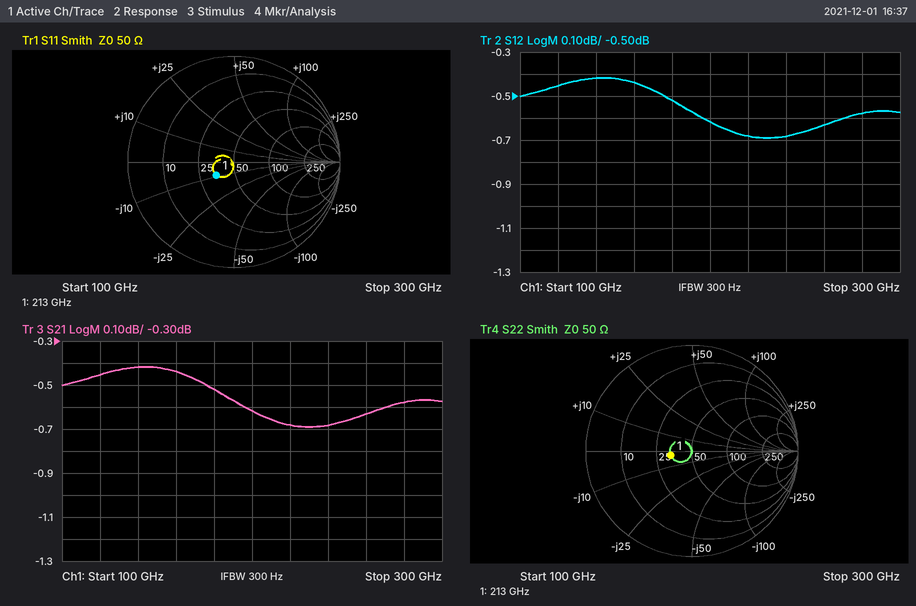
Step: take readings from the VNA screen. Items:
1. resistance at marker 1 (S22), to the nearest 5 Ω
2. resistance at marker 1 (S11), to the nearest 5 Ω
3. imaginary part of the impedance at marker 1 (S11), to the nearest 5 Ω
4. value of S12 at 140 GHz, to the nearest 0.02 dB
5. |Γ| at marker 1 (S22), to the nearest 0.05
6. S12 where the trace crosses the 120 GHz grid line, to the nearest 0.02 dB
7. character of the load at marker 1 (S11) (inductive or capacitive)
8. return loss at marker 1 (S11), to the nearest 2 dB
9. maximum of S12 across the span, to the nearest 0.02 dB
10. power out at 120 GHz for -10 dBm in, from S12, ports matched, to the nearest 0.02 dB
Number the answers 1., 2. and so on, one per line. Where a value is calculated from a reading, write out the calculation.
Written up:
1. 35 Ω
2. 35 Ω
3. -10 Ω
4. -0.42 dB
5. 0.20
6. -0.46 dB
7. capacitive
8. 14 dB
9. -0.42 dB
10. -10 dBm + (-0.46 dB) = -10.46 dBm
